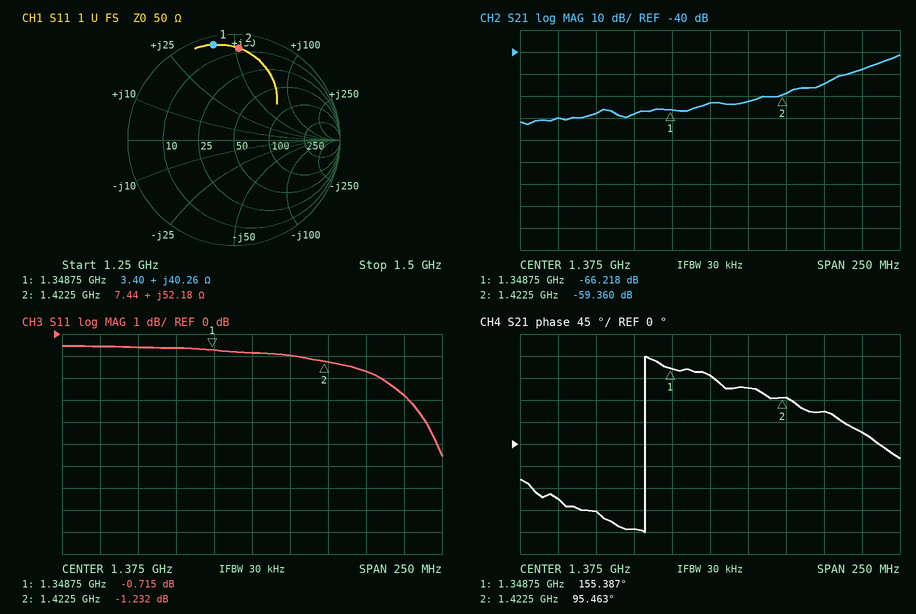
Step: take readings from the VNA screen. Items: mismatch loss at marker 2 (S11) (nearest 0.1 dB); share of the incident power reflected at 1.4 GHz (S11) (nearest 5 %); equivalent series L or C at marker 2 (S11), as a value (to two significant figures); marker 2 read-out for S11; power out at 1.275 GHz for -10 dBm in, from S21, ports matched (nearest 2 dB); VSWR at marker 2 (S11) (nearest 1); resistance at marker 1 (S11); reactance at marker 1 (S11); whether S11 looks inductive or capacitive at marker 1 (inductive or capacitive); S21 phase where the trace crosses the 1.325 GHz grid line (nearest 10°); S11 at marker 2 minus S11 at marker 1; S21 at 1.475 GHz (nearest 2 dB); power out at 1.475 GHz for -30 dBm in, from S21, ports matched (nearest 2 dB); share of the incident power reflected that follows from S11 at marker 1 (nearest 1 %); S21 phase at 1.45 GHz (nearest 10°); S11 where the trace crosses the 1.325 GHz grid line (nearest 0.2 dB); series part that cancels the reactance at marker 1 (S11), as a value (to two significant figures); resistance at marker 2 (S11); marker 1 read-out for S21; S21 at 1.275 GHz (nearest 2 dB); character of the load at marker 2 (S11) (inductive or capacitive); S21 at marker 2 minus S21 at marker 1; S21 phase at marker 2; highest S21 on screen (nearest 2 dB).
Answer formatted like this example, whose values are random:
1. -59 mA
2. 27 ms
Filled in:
1. 6.1 dB
2. 80 %
3. 5.8 nH
4. -1.232 dB
5. -80 dBm
6. 14
7. 3.40 Ω
8. +40.26 Ω
9. inductive
10. -170°
11. -0.517 dB
12. -48 dB
13. -78 dBm
14. 85 %
15. 70°
16. -0.6 dB
17. 2.9 pF
18. 7.44 Ω
19. -66.218 dB
20. -70 dB
21. inductive
22. 6.858 dB
23. 95.463°
24. -42 dB
